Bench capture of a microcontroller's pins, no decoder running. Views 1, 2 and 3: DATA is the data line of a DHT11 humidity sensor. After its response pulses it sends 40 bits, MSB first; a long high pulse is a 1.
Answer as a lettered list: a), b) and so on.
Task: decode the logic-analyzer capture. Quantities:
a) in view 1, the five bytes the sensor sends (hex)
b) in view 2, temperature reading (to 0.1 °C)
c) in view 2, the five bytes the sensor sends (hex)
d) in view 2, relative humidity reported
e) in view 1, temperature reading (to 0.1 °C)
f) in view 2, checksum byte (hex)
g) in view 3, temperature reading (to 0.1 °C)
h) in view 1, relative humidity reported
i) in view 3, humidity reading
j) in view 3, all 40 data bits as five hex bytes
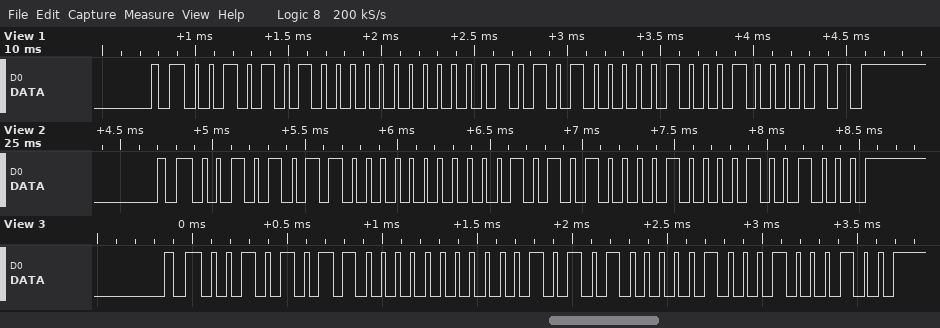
a) 2A 00 15 04 43
b) 21.8 °C
c) 2B 00 15 08 48
d) 43 %
e) 21.4 °C
f) 0x48
g) 21.4 °C
h) 42 %
i) 43 %
j) 2B 00 15 04 44
